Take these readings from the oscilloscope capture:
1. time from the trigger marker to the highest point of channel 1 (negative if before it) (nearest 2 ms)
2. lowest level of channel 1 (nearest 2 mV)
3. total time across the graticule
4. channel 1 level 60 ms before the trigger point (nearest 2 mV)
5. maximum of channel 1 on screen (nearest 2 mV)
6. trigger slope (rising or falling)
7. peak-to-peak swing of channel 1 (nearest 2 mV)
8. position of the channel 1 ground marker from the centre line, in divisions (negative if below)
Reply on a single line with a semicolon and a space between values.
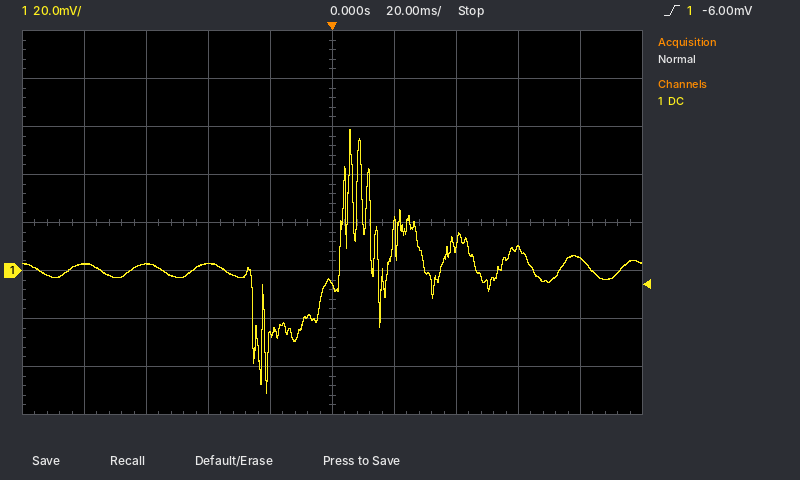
+6 ms; -52 mV; 200 ms; 2 mV; 58 mV; rising; 110 mV; -1.0 div
